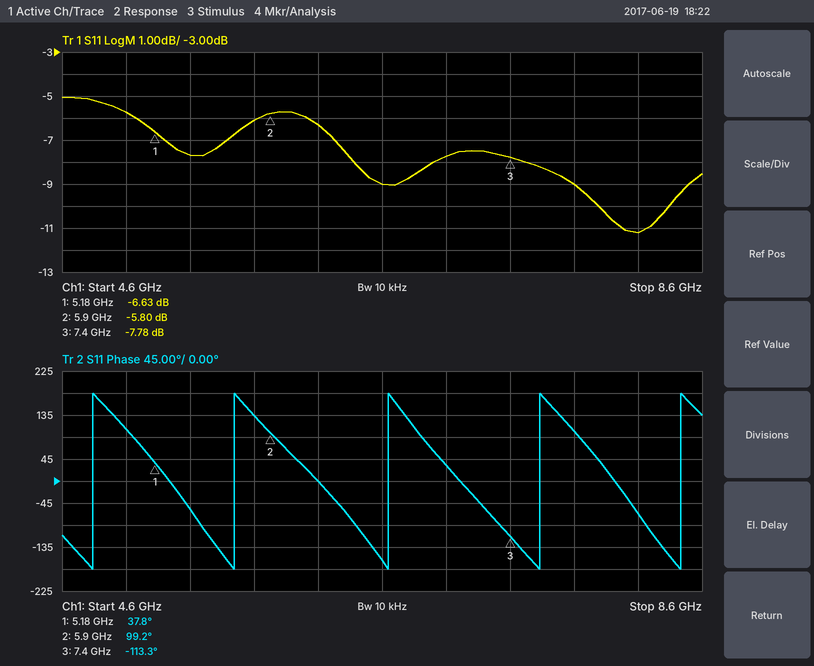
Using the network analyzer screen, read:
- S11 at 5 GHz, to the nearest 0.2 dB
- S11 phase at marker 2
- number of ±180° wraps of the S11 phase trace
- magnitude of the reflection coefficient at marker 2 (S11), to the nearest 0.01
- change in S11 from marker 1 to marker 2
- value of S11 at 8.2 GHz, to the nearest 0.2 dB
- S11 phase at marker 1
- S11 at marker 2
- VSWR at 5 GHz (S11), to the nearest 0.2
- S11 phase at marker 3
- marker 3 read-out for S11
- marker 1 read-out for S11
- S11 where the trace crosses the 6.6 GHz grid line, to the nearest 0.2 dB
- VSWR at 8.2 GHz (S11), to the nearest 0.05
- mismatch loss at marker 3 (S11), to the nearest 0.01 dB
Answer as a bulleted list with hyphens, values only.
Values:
- -5.8 dB
- 99.2°
- 5
- 0.51
- 0.83 dB
- -11.2 dB
- 37.8°
- -5.80 dB
- 3.2
- -113.3°
- -7.78 dB
- -6.63 dB
- -9.0 dB
- 1.75
- 0.79 dB
